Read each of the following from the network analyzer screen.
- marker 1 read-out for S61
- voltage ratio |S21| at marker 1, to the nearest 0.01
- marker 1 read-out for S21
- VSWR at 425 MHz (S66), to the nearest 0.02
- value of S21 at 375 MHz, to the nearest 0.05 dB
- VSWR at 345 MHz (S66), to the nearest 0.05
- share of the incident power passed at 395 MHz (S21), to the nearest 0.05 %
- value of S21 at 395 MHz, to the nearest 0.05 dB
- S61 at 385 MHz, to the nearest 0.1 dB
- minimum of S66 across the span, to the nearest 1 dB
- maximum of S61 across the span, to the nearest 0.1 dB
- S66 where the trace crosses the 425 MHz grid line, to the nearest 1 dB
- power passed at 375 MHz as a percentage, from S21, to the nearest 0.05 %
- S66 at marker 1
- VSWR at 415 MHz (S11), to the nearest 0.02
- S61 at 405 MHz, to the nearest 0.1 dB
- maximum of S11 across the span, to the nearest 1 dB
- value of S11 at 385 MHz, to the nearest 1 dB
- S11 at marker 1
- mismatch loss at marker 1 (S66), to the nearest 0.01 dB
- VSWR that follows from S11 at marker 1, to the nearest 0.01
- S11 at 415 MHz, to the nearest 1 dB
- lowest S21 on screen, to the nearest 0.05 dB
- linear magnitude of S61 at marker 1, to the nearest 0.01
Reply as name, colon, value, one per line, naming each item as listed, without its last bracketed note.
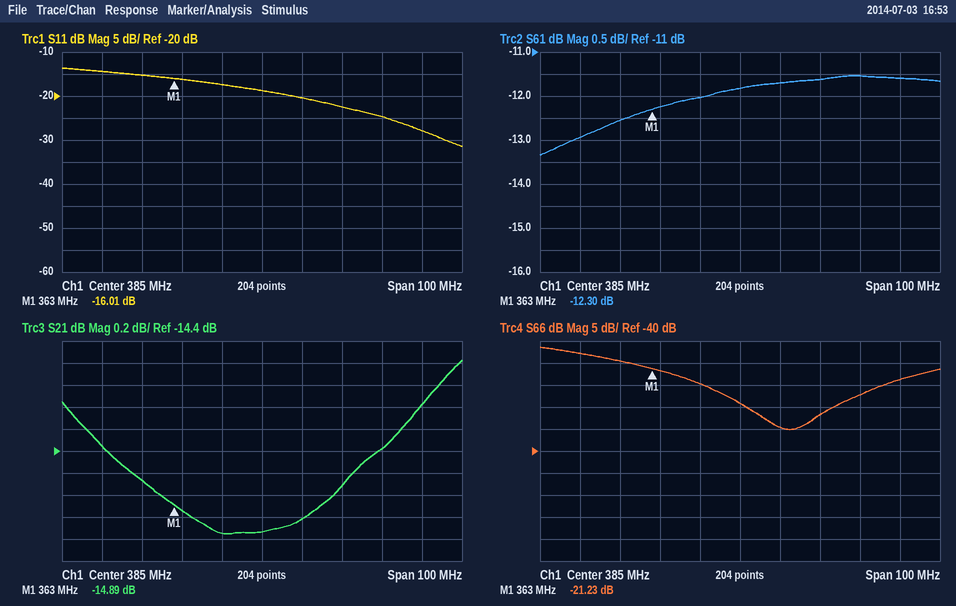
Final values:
marker 1 read-out for S61: -12.30 dB
voltage ratio |S21| at marker 1, to the nearest 0.01: 0.18
marker 1 read-out for S21: -14.89 dB
VSWR at 425 MHz (S66), to the nearest 0.02: 1.14
value of S21 at 375 MHz, to the nearest 0.05 dB: -15.15 dB
VSWR at 345 MHz (S66), to the nearest 0.05: 1.30
share of the incident power passed at 395 MHz (S21), to the nearest 0.05 %: 3.15 %
value of S21 at 395 MHz, to the nearest 0.05 dB: -15.00 dB
S61 at 385 MHz, to the nearest 0.1 dB: -11.8 dB
minimum of S66 across the span, to the nearest 1 dB: -35 dB
maximum of S61 across the span, to the nearest 0.1 dB: -11.5 dB
S66 where the trace crosses the 425 MHz grid line, to the nearest 1 dB: -24 dB
power passed at 375 MHz as a percentage, from S21, to the nearest 0.05 %: 3.05 %
S66 at marker 1: -21.23 dB
VSWR at 415 MHz (S11), to the nearest 0.02: 1.12
S61 at 405 MHz, to the nearest 0.1 dB: -11.6 dB
maximum of S11 across the span, to the nearest 1 dB: -14 dB
value of S11 at 385 MHz, to the nearest 1 dB: -19 dB
S11 at marker 1: -16.01 dB
mismatch loss at marker 1 (S66), to the nearest 0.01 dB: 0.03 dB
VSWR that follows from S11 at marker 1, to the nearest 0.01: 1.38
S11 at 415 MHz, to the nearest 1 dB: -25 dB
lowest S21 on screen, to the nearest 0.05 dB: -15.15 dB
linear magnitude of S61 at marker 1, to the nearest 0.01: 0.24
